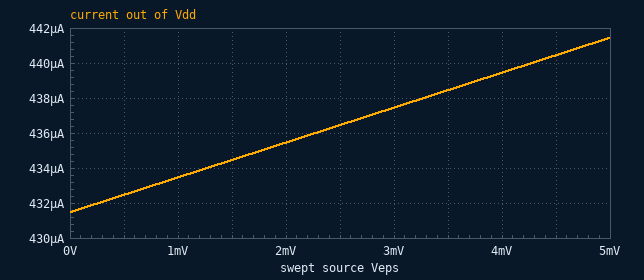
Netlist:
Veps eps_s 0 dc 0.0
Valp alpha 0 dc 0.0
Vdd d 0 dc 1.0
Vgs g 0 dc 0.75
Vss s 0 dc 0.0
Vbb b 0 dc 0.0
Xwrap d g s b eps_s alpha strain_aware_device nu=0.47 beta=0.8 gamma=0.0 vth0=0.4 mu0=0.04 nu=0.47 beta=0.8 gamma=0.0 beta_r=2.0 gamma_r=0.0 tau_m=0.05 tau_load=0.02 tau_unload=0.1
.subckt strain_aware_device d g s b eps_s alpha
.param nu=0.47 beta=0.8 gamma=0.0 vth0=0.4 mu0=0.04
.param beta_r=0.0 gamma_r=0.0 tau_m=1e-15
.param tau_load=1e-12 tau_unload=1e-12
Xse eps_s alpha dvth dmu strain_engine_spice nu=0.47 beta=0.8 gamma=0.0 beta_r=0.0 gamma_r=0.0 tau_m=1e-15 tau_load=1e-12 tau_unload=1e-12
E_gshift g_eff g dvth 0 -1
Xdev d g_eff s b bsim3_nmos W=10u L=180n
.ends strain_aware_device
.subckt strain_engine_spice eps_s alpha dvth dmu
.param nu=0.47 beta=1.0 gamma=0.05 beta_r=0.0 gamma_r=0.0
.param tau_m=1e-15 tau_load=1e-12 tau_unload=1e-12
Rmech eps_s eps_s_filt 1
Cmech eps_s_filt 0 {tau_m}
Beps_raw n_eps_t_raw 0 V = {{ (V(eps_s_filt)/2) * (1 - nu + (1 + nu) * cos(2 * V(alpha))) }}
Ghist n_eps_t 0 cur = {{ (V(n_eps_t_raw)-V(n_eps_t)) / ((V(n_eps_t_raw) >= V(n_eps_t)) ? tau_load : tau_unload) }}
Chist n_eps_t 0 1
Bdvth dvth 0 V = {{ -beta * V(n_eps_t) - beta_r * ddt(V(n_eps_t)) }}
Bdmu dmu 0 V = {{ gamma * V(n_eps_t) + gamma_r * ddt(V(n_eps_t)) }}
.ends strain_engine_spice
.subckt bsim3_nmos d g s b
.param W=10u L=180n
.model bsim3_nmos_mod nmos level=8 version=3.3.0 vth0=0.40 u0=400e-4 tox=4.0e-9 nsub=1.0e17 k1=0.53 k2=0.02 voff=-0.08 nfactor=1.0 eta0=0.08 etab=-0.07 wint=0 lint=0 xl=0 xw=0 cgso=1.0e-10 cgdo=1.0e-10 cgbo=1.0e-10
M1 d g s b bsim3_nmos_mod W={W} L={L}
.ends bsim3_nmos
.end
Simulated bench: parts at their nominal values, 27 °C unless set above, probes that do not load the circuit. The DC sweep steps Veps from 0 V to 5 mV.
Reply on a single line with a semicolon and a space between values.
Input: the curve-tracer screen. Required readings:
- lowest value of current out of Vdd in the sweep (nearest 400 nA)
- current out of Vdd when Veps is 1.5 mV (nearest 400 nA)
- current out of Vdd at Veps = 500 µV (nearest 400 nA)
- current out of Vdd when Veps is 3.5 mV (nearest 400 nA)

431.6 µA; 434.4 µA; 432.4 µA; 438.4 µA
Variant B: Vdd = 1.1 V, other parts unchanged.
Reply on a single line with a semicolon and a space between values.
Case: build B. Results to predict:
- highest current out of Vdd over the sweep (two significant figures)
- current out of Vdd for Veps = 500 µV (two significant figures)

460 µA; 450 µA
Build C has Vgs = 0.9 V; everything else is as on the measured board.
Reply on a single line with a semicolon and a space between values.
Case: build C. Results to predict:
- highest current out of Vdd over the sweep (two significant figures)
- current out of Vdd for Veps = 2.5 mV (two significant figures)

850 µA; 840 µA
